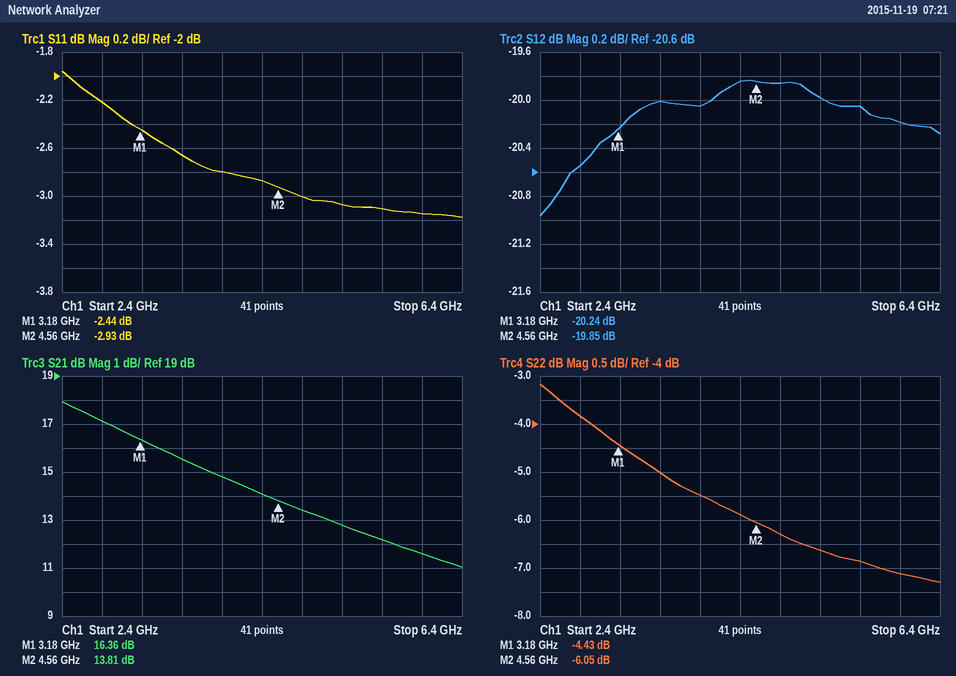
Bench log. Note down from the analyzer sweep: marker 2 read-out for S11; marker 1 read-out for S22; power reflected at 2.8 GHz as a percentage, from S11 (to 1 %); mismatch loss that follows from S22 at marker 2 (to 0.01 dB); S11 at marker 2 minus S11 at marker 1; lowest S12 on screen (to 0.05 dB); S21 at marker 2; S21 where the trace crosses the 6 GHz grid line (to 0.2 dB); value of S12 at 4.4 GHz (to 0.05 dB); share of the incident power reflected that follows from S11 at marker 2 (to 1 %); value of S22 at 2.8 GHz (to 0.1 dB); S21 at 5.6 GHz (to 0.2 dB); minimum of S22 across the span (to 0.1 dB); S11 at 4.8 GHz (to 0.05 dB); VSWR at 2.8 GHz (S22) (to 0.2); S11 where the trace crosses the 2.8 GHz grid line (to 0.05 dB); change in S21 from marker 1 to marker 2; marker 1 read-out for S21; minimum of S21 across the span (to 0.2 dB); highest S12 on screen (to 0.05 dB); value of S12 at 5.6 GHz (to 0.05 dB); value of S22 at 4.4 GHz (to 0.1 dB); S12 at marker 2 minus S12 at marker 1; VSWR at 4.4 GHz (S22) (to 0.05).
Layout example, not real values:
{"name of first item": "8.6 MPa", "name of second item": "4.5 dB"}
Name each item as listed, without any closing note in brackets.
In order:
{"marker 2 read-out for S11": "-2.93 dB", "marker 1 read-out for S22": "-4.43 dB", "power reflected at 2.8 GHz as a percentage, from S11": "60 %", "mismatch loss that follows from S22 at marker 2": "1.24 dB", "S11 at marker 2 minus S11 at marker 1": "-0.49 dB", "lowest S12 on screen": "-20.95 dB", "S21 at marker 2": "13.81 dB", "S21 where the trace crosses the 6 GHz grid line": "11.6 dB", "value of S12 at 4.4 GHz": "-19.85 dB", "share of the incident power reflected that follows from S11 at marker 2": "51 %", "value of S22 at 2.8 GHz": "-3.8 dB", "S21 at 5.6 GHz": "12.2 dB", "minimum of S22 across the span": "-7.3 dB", "S11 at 4.8 GHz": "-3.00 dB", "VSWR at 2.8 GHz (S22)": "4.6", "S11 where the trace crosses the 2.8 GHz grid line": "-2.20 dB", "change in S21 from marker 1 to marker 2": "-2.55 dB", "marker 1 read-out for S21": "16.36 dB", "minimum of S21 across the span": "11.0 dB", "highest S12 on screen": "-19.85 dB", "value of S12 at 5.6 GHz": "-20.05 dB", "value of S22 at 4.4 GHz": "-5.9 dB", "S12 at marker 2 minus S12 at marker 1": "0.39 dB", "VSWR at 4.4 GHz (S22)": "3.05"}
